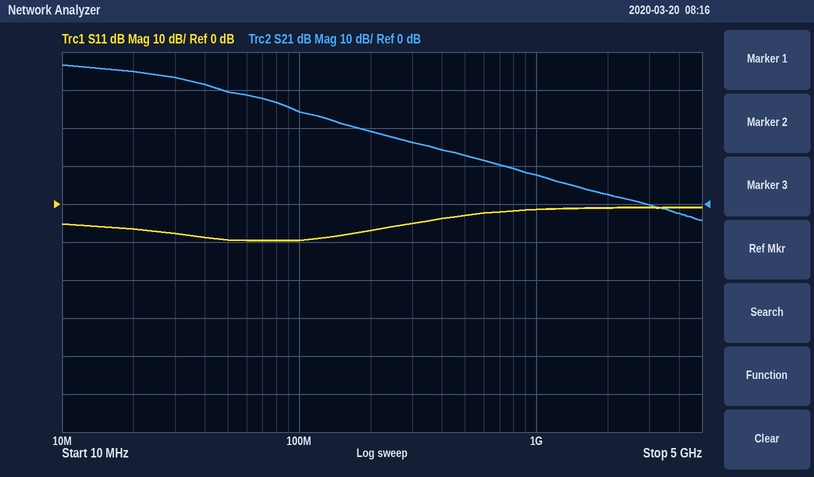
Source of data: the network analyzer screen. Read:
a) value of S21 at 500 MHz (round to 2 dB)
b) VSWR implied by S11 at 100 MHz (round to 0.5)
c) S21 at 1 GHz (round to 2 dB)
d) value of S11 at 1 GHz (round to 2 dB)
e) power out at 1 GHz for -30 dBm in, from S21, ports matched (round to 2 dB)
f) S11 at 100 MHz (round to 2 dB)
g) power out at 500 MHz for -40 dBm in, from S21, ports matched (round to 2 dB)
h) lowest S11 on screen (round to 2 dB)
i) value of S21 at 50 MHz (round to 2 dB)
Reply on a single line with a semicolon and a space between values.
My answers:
12 dB; 2.0; 8 dB; -2 dB; -22 dBm; -10 dB; -28 dBm; -10 dB; 30 dB
